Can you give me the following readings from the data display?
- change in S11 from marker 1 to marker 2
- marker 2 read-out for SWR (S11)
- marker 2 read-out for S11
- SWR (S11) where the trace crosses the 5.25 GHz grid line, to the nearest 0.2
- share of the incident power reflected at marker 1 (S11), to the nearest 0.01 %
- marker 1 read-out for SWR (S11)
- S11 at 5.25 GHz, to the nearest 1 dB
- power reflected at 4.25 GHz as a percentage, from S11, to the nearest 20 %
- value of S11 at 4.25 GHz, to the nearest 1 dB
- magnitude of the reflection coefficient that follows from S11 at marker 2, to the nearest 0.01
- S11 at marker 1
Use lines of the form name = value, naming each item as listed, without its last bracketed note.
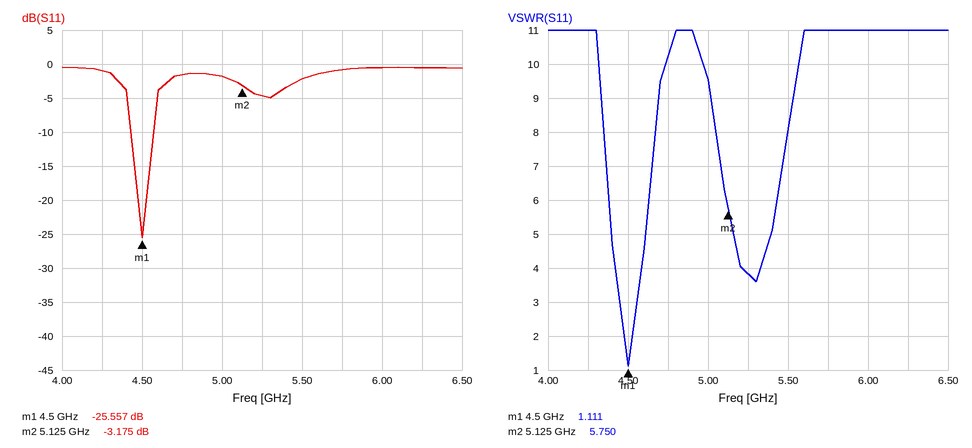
change in S11 from marker 1 to marker 2 = 22.382 dB
marker 2 read-out for SWR = 5.750
marker 2 read-out for S11 = -3.175 dB
SWR (S11) where the trace crosses the 5.25 GHz grid line, to the nearest 0.2 = 3.8
share of the incident power reflected at marker 1 (S11), to the nearest 0.01 % = 0.28 %
marker 1 read-out for SWR = 1.111
S11 at 5.25 GHz, to the nearest 1 dB = -5 dB
power reflected at 4.25 GHz as a percentage, from S11, to the nearest 20 % = 80 %
value of S11 at 4.25 GHz, to the nearest 1 dB = -1 dB
magnitude of the reflection coefficient that follows from S11 at marker 2, to the nearest 0.01 = 0.69
S11 at marker 1 = -25.557 dB
